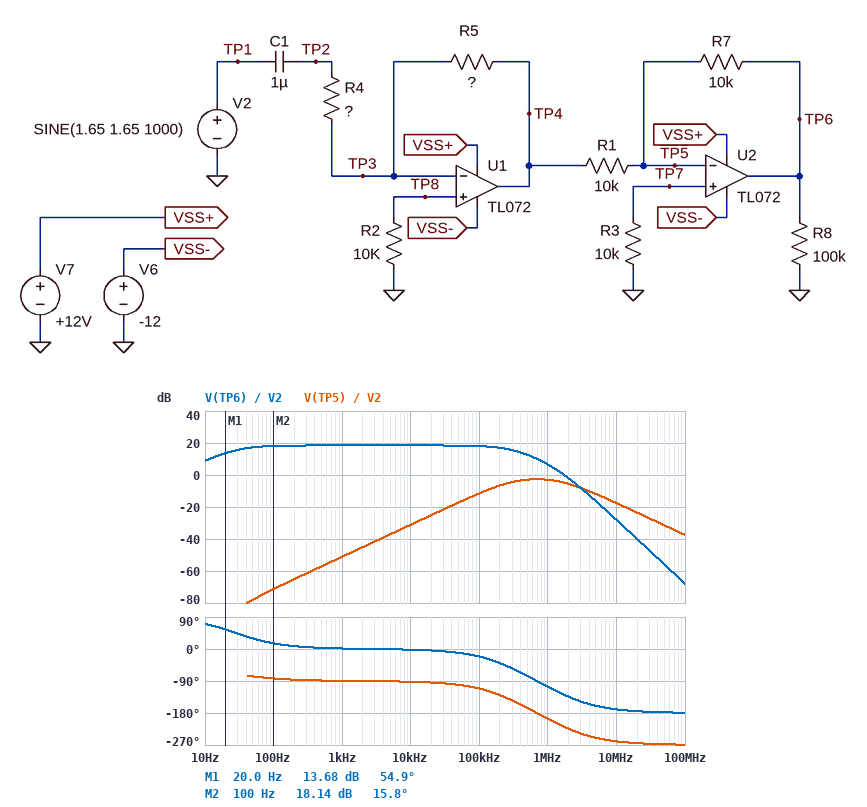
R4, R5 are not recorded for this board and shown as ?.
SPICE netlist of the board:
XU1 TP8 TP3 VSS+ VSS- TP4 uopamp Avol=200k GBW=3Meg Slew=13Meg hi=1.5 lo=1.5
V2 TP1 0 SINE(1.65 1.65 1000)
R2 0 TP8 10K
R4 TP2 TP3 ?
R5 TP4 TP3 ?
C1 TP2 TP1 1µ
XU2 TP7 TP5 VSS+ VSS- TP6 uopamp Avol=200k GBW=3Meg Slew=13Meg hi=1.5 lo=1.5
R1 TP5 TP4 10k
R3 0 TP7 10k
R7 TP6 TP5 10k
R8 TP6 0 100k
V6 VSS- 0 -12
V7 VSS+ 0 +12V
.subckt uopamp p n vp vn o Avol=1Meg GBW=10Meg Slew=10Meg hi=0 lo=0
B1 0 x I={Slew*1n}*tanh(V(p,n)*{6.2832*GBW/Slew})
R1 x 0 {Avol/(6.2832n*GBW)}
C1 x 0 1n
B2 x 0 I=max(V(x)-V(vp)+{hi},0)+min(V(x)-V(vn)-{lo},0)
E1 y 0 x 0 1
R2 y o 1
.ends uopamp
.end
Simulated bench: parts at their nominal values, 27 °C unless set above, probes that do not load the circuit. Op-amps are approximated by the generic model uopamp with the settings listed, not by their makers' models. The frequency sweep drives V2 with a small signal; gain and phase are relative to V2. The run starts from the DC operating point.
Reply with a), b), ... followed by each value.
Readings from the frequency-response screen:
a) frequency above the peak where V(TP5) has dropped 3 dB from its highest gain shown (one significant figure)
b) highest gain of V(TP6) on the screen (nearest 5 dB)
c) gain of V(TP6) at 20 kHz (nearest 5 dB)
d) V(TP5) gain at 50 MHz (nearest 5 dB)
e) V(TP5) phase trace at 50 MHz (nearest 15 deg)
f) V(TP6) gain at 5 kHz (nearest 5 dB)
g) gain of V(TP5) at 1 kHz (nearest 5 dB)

a) 2 MHz
b) 20 dB
c) 20 dB
d) -30 dB
e) -270 deg
f) 20 dB
g) -50 dB
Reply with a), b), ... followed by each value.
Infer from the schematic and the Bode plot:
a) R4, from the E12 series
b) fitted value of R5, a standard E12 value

a) 5.6 kΩ
b) 47 kΩ
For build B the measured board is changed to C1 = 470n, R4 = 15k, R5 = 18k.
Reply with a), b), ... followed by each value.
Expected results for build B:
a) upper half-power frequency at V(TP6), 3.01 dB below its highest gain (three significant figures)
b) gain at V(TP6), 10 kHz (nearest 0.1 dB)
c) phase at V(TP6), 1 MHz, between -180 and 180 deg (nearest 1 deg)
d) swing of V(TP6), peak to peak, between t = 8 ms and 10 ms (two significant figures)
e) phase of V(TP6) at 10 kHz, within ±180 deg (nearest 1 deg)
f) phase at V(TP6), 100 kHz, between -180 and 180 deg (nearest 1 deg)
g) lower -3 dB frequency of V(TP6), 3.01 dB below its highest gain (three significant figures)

a) 919 kHz
b) 1.6 dB
c) -70 deg
d) 4.0 V
e) -1 deg
f) -8 deg
g) 22.6 Hz
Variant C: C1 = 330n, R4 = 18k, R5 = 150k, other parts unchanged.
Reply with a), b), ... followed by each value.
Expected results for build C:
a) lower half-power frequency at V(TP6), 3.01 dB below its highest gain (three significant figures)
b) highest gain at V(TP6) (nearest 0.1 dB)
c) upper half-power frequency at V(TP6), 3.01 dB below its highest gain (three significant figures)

a) 26.8 Hz
b) 18.4 dB
c) 308 kHz
